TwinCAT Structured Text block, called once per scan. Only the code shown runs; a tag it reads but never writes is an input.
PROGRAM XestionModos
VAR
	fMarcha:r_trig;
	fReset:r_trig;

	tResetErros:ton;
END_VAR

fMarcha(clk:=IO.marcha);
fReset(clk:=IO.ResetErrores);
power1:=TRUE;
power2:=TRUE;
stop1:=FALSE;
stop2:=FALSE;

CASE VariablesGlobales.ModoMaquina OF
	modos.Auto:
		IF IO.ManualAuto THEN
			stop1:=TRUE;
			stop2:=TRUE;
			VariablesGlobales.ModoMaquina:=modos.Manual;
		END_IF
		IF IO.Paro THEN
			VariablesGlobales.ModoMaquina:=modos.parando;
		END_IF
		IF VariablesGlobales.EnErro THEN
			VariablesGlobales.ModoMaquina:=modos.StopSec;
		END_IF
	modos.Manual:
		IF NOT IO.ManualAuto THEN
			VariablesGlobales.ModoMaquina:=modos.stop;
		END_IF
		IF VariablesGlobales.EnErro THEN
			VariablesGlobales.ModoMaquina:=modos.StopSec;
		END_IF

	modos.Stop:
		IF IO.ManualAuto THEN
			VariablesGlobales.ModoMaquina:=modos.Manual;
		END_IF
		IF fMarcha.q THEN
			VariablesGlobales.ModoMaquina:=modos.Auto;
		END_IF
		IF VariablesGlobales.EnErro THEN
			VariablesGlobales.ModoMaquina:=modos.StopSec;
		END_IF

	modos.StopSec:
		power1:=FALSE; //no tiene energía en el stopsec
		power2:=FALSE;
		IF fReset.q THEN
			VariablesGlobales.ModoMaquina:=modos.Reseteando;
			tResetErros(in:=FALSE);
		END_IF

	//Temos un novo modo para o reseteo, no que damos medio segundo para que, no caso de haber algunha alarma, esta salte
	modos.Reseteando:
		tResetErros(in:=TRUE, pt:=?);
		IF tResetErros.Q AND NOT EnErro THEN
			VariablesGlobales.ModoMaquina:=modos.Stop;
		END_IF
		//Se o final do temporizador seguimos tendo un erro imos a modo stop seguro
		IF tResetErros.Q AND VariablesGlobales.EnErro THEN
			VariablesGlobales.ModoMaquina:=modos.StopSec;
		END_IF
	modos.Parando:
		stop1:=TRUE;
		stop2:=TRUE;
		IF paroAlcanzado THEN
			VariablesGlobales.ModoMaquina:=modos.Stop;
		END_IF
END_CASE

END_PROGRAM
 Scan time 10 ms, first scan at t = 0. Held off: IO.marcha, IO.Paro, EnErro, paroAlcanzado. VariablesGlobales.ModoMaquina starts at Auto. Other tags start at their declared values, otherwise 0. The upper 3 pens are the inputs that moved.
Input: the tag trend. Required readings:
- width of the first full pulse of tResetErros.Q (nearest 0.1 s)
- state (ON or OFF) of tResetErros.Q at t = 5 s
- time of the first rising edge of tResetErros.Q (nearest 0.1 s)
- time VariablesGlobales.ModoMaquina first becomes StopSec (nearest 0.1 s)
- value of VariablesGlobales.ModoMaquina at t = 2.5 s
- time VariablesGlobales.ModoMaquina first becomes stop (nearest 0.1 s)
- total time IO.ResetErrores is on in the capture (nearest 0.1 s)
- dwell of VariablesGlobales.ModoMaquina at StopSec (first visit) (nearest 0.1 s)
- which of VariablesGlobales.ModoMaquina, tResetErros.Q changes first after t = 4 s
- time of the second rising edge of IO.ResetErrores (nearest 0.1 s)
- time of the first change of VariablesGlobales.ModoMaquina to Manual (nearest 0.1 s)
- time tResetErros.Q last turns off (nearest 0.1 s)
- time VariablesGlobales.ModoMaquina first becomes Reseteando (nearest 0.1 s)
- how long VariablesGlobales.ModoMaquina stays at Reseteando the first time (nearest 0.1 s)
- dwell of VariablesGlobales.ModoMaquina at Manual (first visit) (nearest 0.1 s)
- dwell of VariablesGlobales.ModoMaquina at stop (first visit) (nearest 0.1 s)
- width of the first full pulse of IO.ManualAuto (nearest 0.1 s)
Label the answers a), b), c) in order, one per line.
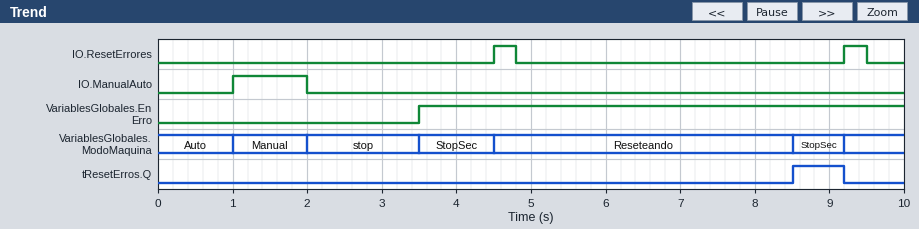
a) 0.7 s
b) OFF
c) 8.5 s
d) 3.5 s
e) stop
f) 2.0 s
g) 0.6 s
h) 1.0 s
i) VariablesGlobales.ModoMaquina
j) 9.2 s
k) 1.0 s
l) 9.2 s
m) 4.5 s
n) 4.0 s
o) 1.0 s
p) 1.5 s
q) 1.0 s
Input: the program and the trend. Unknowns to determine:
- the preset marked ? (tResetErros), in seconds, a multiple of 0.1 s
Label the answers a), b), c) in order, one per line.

a) 4.0 s
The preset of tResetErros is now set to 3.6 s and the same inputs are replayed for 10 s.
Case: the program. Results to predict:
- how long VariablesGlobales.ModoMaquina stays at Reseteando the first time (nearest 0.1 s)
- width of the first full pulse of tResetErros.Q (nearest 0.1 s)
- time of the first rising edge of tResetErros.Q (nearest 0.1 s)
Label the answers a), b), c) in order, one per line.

a) 3.6 s
b) 1.1 s
c) 8.1 s
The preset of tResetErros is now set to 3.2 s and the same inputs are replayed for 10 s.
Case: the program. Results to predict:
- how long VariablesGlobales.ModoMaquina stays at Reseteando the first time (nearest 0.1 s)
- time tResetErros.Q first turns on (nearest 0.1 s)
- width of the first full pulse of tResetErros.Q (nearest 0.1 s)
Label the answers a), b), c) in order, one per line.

a) 3.2 s
b) 7.7 s
c) 1.5 s
